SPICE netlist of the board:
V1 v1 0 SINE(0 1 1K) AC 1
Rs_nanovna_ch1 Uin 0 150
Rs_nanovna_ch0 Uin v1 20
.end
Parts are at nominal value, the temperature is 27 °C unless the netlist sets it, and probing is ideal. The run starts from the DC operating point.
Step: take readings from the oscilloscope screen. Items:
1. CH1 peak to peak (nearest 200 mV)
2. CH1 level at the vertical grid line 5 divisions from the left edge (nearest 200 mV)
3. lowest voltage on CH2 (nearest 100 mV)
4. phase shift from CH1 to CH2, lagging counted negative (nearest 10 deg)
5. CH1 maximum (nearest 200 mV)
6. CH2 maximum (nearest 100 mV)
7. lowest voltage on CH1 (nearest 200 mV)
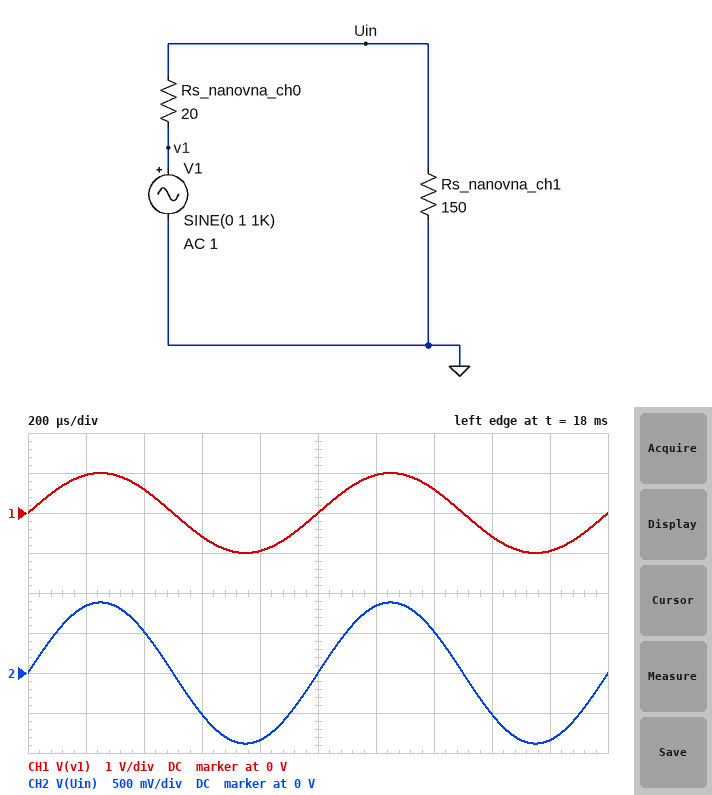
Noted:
2.0 V
0 V
-900 mV
0 deg
1.0 V
900 mV
-1.0 V
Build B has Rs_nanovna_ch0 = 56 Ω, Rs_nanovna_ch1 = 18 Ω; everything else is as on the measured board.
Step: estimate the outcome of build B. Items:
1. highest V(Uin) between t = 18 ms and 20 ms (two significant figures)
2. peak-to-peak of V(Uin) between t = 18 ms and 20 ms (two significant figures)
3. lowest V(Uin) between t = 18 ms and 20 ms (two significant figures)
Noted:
240 mV
490 mV
-240 mV
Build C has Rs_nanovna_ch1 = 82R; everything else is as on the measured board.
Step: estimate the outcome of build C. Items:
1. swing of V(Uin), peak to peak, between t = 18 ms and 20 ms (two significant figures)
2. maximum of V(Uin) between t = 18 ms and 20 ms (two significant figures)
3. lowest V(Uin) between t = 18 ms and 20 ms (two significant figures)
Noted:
1.6 V
800 mV
-800 mV
